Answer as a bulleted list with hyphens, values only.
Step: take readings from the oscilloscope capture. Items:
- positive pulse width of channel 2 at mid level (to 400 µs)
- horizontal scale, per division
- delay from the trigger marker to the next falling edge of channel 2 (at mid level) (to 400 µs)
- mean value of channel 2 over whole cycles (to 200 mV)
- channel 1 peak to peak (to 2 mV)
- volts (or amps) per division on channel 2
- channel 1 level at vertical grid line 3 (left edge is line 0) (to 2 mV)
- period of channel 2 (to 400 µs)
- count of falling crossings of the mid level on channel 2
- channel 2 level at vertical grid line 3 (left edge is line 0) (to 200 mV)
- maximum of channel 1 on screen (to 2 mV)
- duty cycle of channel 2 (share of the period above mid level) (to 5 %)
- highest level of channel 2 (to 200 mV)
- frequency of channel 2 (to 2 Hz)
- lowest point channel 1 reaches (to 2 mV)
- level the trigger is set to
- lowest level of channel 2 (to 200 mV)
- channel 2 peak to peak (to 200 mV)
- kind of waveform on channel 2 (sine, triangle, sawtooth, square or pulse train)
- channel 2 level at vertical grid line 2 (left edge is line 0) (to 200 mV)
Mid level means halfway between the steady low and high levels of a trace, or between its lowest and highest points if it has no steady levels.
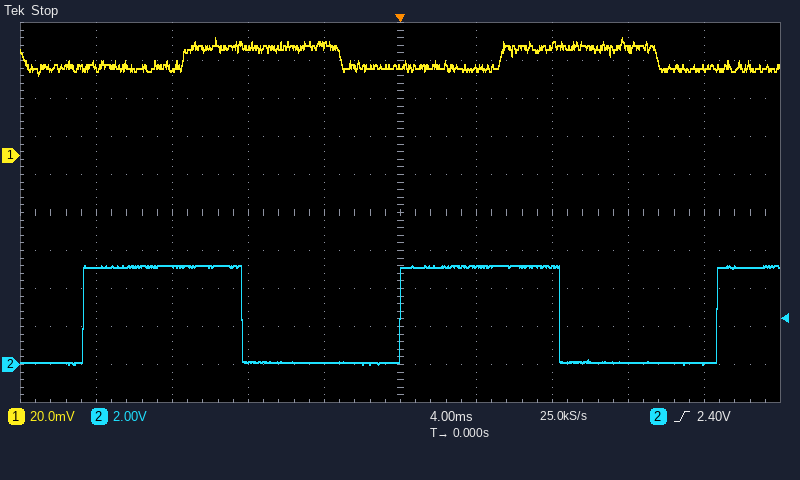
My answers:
- 8.4 ms
- 4 ms
- 8.4 ms
- 2.6 V
- 20 mV
- 2 V
- 58 mV
- 16.8 ms
- 2
- 200 mV
- 62 mV
- 50 %
- 5.2 V
- 60 Hz
- 42 mV
- 2.40 V
- 0.0 V
- 5.2 V
- square
- 5.2 V
